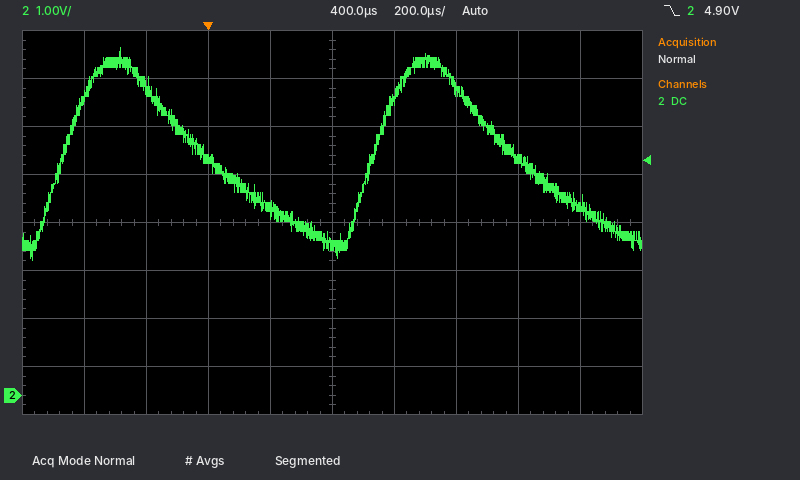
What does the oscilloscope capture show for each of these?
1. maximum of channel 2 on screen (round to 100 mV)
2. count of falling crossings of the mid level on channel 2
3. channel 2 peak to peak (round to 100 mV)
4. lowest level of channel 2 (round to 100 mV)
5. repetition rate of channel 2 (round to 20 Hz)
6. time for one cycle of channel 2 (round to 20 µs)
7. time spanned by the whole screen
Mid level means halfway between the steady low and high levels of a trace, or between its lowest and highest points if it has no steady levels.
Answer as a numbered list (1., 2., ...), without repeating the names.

1. 7.2 V
2. 2
3. 4.4 V
4. 2.8 V
5. 1.00 kHz
6. 1.00 ms
7. 2 ms
